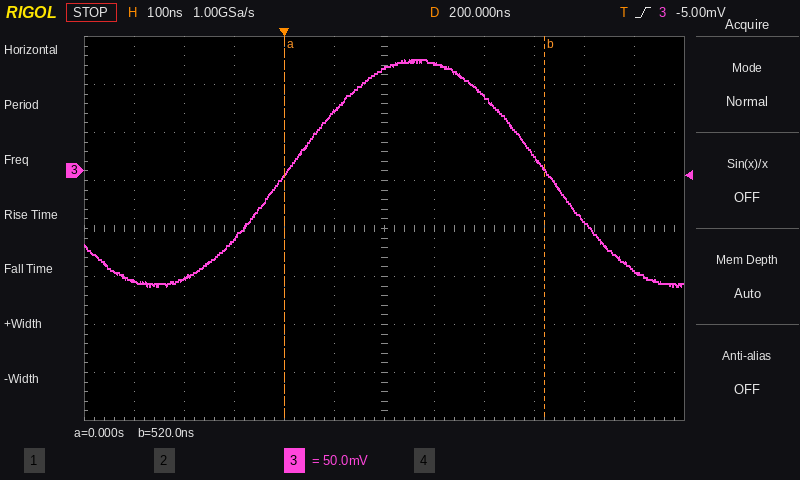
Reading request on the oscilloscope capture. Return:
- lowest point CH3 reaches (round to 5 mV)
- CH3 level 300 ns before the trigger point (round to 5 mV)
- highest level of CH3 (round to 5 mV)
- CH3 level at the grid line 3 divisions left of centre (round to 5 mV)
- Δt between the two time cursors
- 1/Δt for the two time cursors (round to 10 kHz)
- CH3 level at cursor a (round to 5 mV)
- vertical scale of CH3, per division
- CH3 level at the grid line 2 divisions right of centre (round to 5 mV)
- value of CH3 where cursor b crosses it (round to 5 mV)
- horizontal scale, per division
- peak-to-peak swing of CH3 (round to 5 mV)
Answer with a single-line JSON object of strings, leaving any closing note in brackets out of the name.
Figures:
{"lowest point CH3 reaches": "-120 mV", "CH3 level 300 ns before the trigger point": "-115 mV", "highest level of CH3": "115 mV", "CH3 level at the grid line 3 divisions left of centre": "-70 mV", "Δt between the two time cursors": "520 ns", "1/Δt for the two time cursors": "1.92 MHz", "CH3 level at cursor a": "-5 mV", "vertical scale of CH3, per division": "50 mV", "CH3 level at the grid line 2 divisions right of centre": "80 mV", "value of CH3 where cursor b crosses it": "0 mV", "horizontal scale, per division": "100 ns", "peak-to-peak swing of CH3": "235 mV"}
